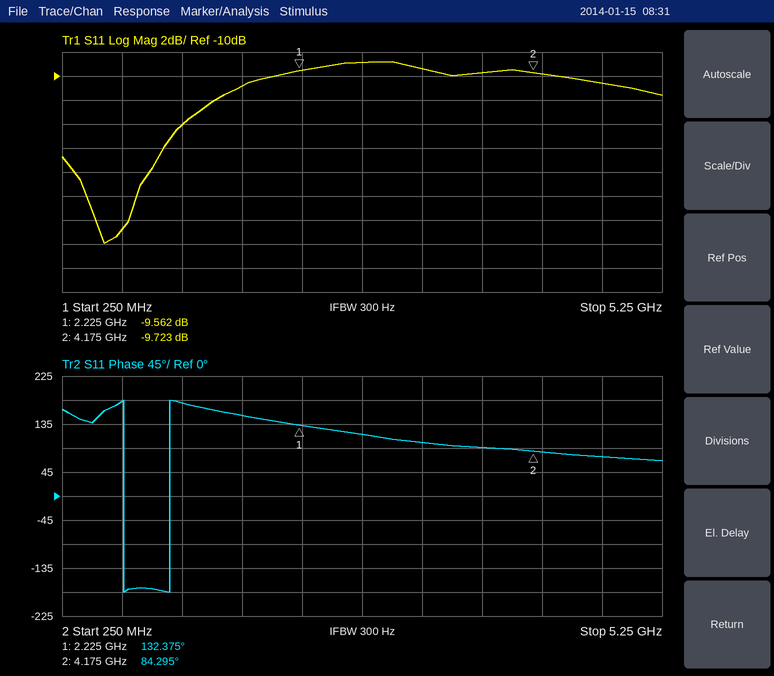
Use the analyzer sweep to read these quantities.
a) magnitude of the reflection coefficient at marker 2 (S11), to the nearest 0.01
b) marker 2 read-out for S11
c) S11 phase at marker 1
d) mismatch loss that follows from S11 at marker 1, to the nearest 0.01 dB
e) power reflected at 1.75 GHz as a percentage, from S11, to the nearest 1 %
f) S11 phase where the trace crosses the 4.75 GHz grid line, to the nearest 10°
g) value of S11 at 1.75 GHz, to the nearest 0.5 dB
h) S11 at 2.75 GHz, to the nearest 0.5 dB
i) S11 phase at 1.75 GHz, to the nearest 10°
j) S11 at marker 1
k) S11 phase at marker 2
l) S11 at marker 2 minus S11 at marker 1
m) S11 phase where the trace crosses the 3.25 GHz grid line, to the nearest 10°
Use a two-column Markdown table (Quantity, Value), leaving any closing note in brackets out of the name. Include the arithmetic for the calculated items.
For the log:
| Quantity | Value |
|---|---|
| magnitude of the reflection coefficient at marker 2 (S11), to the nearest 0.01 | 10^(-9.723/20) ≈ 0.33 |
| marker 2 read-out for S11 | -9.723 dB |
| S11 phase at marker 1 | 132.375° |
| mismatch loss that follows from S11 at marker 1, to the nearest 0.01 dB | −10 log10(1 − 10^(-9.562/10)) ≈ 0.51 dB |
| power reflected at 1.75 GHz as a percentage, from S11, to the nearest 1 % | 10^(-11/10) ≈ 8 % |
| S11 phase where the trace crosses the 4.75 GHz grid line, to the nearest 10° | 70° |
| value of S11 at 1.75 GHz, to the nearest 0.5 dB | -11.0 dB |
| S11 at 2.75 GHz, to the nearest 0.5 dB | -9.0 dB |
| S11 phase at 1.75 GHz, to the nearest 10° | 150° |
| S11 at marker 1 | -9.562 dB |
| S11 phase at marker 2 | 84.295° |
| S11 at marker 2 minus S11 at marker 1 | -9.723 − (-9.562) = -0.161 dB |
| S11 phase where the trace crosses the 3.25 GHz grid line, to the nearest 10° | 100° |
